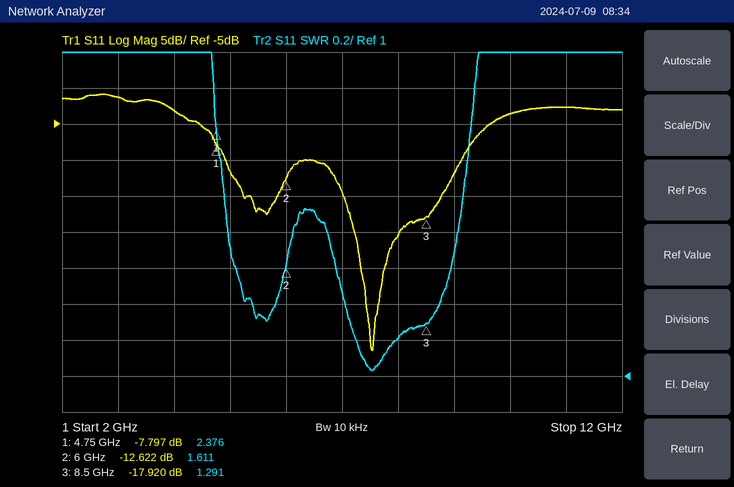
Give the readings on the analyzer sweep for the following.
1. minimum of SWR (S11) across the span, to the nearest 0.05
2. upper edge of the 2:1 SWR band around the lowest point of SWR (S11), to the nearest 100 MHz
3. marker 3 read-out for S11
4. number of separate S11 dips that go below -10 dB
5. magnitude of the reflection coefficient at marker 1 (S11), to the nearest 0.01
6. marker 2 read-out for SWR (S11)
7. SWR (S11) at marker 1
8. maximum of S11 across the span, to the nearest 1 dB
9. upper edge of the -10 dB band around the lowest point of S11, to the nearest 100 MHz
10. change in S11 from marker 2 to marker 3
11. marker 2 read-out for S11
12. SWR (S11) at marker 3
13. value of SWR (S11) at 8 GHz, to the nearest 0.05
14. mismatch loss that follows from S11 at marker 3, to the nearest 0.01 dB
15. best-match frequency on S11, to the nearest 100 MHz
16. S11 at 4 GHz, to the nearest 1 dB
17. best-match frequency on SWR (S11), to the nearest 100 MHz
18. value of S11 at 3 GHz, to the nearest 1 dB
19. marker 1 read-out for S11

1.05
9.2 GHz
-17.920 dB
2
0.41
1.611
2.376
-1 dB
9.1 GHz
-5.298 dB
-12.622 dB
1.291
1.20
0.07 dB
7.5 GHz
-3 dB
7.5 GHz
-1 dB
-7.797 dB
